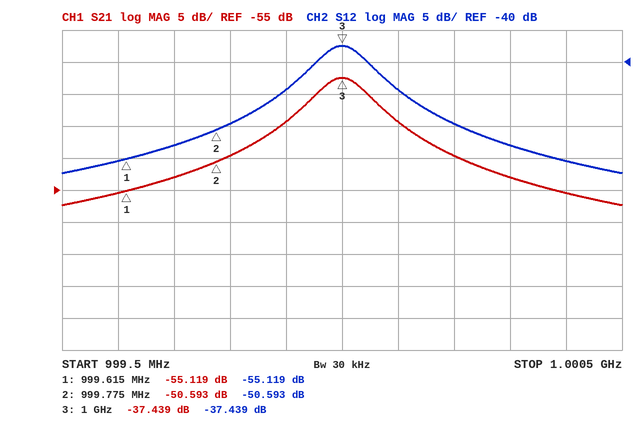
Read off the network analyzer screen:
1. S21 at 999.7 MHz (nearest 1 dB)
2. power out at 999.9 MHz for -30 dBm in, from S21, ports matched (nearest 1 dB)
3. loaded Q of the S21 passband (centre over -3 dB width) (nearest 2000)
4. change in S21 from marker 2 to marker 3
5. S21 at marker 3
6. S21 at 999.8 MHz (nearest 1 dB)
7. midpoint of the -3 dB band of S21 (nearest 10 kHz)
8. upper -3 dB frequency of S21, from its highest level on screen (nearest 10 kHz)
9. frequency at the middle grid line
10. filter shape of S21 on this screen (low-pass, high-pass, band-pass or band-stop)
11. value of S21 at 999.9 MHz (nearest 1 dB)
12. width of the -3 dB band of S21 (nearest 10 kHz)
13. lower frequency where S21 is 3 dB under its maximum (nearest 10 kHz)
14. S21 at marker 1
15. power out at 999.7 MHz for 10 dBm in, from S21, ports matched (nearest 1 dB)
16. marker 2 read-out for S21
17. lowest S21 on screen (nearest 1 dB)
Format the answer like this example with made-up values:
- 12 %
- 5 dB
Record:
- -53 dB
- -74 dBm
- 10000
- 13.154 dB
- -37.439 dB
- -50 dB
- 1.00000 GHz
- 1.00005 GHz
- 1 GHz
- band-pass
- -44 dB
- 100 kHz
- 999.95 MHz
- -55.119 dB
- -43 dBm
- -50.593 dB
- -57 dB
